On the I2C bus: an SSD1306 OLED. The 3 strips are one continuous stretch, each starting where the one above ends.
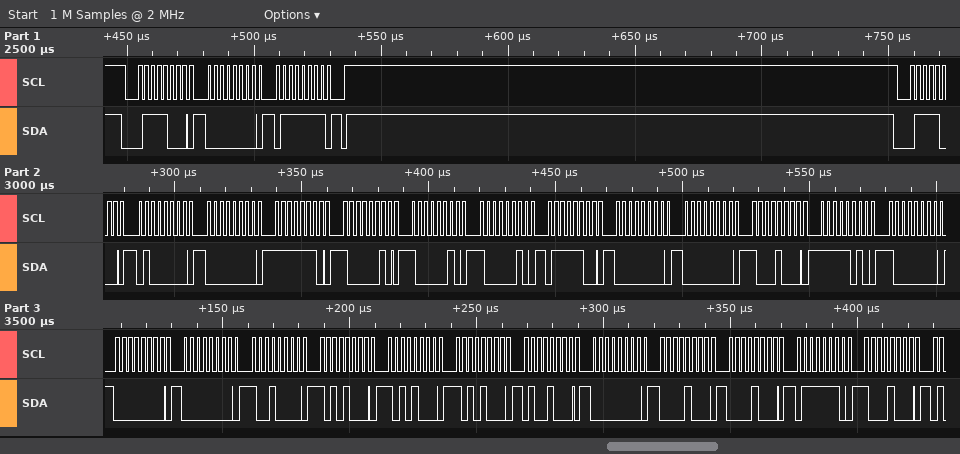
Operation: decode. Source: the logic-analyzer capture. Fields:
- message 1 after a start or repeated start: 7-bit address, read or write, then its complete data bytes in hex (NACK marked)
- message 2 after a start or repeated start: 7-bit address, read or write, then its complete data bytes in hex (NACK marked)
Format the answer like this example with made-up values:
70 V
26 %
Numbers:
0x3C write: 00 7F
0x3C write: 40 00 FE 82 82 82 7C 00 00 88 FA 80 00 00 90 A8 A8 A8 48 00 08 08 7E 88
